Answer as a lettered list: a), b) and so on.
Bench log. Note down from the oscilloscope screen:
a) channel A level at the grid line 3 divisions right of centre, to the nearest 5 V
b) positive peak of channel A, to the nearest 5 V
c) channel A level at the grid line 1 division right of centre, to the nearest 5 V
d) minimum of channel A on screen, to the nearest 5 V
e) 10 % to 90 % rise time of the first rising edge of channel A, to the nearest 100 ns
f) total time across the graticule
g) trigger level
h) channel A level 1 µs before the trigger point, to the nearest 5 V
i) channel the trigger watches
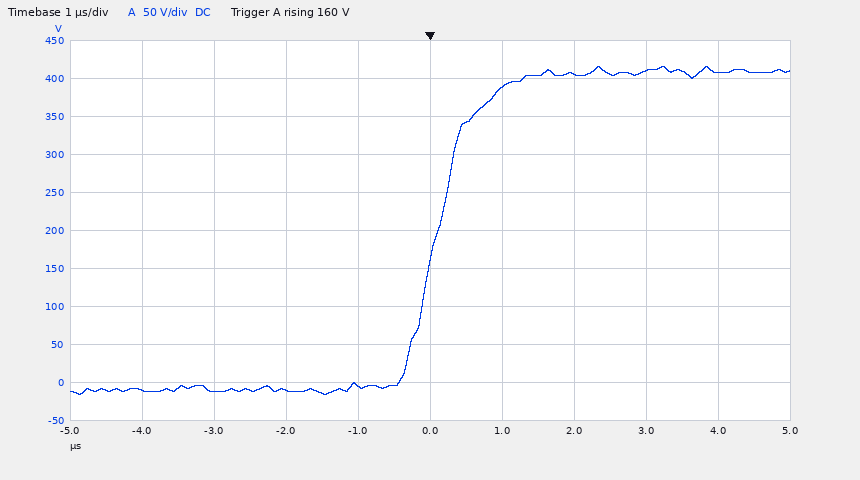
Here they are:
a) 410 V
b) 415 V
c) 390 V
d) -15 V
e) 1.1 µs
f) 10 µs
g) 160 V
h) -5 V
i) channel A
